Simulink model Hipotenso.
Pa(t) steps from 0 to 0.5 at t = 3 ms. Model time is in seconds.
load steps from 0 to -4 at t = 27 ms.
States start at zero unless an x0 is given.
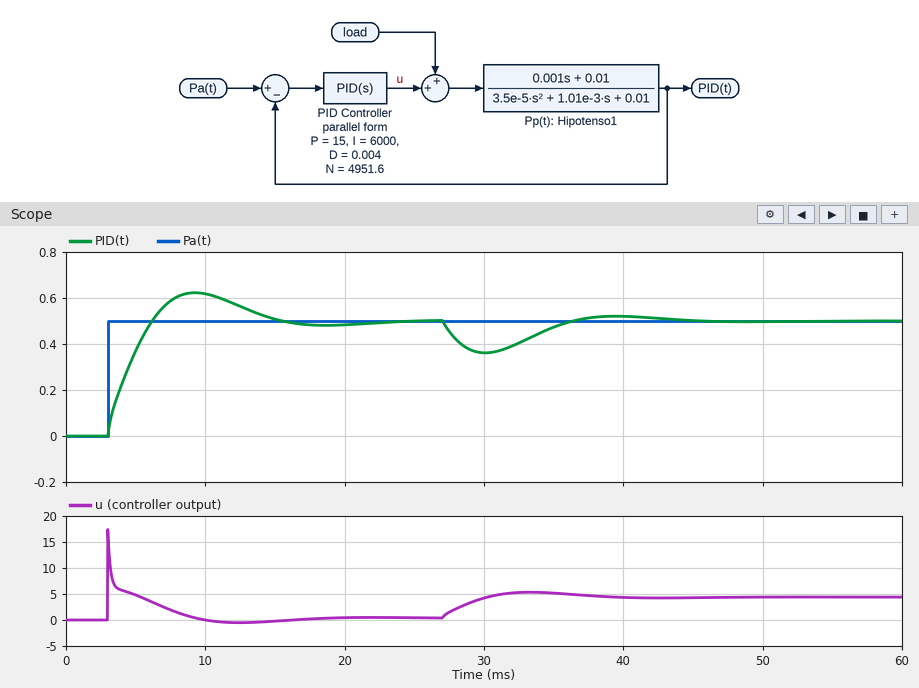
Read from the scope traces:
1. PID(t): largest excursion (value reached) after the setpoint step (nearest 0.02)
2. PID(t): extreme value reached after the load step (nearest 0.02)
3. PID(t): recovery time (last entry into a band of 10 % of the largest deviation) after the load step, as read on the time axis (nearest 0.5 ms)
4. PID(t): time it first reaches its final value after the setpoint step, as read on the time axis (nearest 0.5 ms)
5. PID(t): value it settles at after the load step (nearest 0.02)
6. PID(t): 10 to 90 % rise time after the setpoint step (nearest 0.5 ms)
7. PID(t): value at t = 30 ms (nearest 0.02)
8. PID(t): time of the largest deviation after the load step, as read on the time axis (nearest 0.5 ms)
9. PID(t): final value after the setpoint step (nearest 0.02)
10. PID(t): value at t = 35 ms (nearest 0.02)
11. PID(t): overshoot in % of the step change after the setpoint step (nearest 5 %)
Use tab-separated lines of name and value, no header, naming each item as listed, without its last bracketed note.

PID(t): largest excursion (value reached) after the setpoint step	0.62
PID(t): extreme value reached after the load step	0.36
PID(t): recovery time (last entry into a band of 10 % of the largest deviation) after the load step, as read on the time axis	42.0 ms
PID(t): time it first reaches its final value after the setpoint step, as read on the time axis	6.0 ms
PID(t): value it settles at after the load step	0.50
PID(t): 10 to 90 % rise time after the setpoint step	2.5 ms
PID(t): value at t = 30 ms	0.36
PID(t): time of the largest deviation after the load step, as read on the time axis	30.0 ms
PID(t): final value after the setpoint step	0.50
PID(t): value at t = 35 ms	0.48
PID(t): overshoot in % of the step change after the setpoint step	25 %
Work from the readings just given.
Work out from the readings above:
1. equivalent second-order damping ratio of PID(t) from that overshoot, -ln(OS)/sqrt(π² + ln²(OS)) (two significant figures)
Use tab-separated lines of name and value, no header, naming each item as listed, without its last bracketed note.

equivalent second-order damping ratio of PID(t) from that overshoot, -ln(OS)/sqrt(π² + ln²(OS))	0.40
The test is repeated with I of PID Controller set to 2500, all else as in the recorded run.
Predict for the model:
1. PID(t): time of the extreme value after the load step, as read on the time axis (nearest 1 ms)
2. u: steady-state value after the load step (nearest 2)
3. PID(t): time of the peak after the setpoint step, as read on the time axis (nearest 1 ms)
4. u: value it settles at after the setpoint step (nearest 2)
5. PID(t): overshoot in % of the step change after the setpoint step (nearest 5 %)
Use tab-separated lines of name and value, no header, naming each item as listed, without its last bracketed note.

PID(t): time of the extreme value after the load step, as read on the time axis	31 ms
u: steady-state value after the load step	4
PID(t): time of the peak after the setpoint step, as read on the time axis	12 ms
u: value it settles at after the setpoint step	0
PID(t): overshoot in % of the step change after the setpoint step	15 %
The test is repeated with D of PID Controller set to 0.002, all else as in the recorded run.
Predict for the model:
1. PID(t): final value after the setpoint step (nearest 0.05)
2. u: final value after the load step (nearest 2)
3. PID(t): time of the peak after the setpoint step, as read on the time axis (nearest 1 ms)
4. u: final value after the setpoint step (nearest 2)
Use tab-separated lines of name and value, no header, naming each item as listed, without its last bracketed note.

PID(t): final value after the setpoint step	0.50
u: final value after the load step	4
PID(t): time of the peak after the setpoint step, as read on the time axis	9 ms
u: final value after the setpoint step	0
